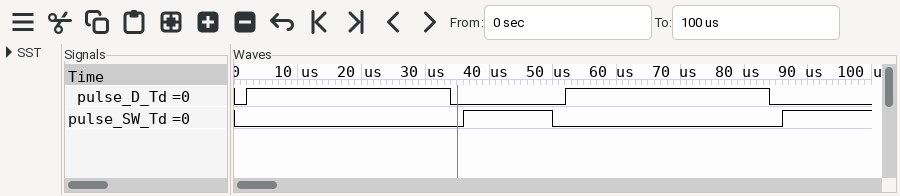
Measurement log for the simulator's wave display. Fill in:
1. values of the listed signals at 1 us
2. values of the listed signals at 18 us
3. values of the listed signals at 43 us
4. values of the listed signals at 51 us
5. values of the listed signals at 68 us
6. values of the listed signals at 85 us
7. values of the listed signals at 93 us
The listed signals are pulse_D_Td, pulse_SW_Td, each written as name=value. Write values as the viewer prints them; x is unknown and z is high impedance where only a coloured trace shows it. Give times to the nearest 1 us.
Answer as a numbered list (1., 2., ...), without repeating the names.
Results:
1. pulse_D_Td=0, pulse_SW_Td=0
2. pulse_D_Td=1, pulse_SW_Td=0
3. pulse_D_Td=0, pulse_SW_Td=1
4. pulse_D_Td=0, pulse_SW_Td=0
5. pulse_D_Td=1, pulse_SW_Td=0
6. pulse_D_Td=0, pulse_SW_Td=0
7. pulse_D_Td=0, pulse_SW_Td=1
